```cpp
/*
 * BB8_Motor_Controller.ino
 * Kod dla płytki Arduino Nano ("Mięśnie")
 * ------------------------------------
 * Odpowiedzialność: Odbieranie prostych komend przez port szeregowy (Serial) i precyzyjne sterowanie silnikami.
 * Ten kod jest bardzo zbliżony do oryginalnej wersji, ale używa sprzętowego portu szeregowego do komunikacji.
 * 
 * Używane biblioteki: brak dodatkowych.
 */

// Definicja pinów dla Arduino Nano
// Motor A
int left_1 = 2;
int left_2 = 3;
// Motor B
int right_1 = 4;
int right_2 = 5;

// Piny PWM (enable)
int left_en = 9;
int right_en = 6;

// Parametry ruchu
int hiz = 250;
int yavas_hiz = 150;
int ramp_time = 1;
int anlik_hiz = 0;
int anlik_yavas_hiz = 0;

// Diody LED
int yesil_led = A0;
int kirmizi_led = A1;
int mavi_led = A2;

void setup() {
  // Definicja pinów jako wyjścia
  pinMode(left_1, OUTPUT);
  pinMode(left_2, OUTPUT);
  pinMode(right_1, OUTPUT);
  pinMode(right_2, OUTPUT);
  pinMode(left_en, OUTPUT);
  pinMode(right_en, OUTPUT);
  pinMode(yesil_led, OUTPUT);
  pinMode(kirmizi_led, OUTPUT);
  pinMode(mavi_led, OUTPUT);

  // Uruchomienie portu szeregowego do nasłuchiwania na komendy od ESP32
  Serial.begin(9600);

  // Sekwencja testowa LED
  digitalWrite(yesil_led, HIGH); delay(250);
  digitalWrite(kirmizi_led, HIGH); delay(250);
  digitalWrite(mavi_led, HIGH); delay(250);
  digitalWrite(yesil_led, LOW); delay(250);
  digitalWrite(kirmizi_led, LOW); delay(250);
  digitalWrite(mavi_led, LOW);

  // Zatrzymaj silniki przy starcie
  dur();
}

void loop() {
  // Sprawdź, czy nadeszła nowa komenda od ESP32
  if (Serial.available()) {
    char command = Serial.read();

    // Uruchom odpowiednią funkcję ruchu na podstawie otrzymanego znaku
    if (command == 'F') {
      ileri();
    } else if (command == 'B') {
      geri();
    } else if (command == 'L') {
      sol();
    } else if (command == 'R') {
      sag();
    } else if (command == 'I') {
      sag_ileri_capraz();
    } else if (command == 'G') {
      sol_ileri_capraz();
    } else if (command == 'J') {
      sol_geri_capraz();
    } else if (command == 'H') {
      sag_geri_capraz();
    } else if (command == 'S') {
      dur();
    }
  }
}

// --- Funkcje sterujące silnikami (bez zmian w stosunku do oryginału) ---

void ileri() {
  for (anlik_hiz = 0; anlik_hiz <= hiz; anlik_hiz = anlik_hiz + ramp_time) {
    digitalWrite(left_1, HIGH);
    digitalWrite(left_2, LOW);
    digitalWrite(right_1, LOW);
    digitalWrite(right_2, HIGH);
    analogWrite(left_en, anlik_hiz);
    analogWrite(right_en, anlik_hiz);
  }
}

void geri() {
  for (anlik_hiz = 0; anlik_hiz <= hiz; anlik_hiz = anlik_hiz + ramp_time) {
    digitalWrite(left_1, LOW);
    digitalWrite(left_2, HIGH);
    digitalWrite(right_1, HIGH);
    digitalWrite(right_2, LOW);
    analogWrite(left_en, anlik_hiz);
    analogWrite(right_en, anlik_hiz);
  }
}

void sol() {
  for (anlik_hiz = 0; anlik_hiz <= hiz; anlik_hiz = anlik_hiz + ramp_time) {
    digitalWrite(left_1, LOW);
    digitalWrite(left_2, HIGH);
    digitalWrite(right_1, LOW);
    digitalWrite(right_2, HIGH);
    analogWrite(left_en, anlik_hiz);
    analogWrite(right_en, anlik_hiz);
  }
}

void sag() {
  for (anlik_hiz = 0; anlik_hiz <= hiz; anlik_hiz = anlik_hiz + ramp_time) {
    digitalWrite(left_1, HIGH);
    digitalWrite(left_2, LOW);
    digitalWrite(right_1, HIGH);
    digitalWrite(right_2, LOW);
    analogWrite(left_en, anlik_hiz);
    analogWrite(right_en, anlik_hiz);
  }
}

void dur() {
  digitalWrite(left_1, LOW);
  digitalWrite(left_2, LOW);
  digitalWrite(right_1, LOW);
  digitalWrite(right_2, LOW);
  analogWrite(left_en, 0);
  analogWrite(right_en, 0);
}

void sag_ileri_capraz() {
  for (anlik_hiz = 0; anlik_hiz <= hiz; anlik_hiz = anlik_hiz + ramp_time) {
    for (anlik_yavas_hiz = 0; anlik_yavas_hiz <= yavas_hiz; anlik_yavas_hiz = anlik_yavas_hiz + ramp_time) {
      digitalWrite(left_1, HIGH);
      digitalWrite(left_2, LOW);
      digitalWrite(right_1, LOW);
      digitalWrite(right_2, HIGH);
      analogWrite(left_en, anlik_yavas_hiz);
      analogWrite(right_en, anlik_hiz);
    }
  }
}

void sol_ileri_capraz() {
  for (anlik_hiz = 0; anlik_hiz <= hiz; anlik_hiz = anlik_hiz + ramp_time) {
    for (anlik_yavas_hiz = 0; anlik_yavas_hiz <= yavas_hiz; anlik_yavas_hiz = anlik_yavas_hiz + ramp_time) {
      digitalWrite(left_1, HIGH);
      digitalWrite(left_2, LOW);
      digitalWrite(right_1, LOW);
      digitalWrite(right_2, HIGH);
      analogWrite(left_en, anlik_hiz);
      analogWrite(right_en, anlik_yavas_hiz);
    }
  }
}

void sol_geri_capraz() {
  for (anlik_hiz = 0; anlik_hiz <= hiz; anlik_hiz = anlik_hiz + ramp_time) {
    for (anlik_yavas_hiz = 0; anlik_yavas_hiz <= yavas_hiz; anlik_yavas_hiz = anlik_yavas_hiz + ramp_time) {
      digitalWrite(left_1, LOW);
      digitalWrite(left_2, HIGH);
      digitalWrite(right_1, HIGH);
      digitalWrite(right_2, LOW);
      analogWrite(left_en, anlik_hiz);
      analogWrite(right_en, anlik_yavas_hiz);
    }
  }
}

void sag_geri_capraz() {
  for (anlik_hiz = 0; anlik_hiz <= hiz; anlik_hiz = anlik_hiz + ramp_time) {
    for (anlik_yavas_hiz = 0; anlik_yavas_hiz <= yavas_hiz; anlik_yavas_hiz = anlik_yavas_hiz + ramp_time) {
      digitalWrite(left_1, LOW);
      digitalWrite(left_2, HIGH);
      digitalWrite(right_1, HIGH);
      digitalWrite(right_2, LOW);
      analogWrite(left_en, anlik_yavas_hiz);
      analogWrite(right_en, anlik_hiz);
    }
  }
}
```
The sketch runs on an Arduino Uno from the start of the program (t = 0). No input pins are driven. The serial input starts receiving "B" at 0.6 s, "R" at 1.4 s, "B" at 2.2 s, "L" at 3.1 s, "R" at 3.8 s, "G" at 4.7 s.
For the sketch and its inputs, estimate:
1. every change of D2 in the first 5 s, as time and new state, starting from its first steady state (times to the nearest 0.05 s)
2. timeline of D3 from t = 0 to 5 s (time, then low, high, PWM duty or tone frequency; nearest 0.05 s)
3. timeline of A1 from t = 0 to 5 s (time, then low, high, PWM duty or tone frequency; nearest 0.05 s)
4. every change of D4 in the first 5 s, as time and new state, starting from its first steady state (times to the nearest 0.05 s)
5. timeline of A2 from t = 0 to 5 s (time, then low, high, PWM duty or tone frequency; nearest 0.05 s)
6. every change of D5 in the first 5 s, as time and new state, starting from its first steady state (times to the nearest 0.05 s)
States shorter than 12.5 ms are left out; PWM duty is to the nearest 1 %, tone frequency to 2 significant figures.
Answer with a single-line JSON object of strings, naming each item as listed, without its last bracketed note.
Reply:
{"every change of D2 in the first 5 s, as time and new state, starting from its first steady state": "0 s low; 1.4 s high; 2.2 s low; 3.8 s high", "timeline of D3 from t = 0 to 5 s": "0 s low; 1.25 s high; 1.4 s low; 2.2 s high; 3.8 s low", "timeline of A1 from t = 0 to 5 s": "0 s low; 0.25 s high; 1 s low", "every change of D4 in the first 5 s, as time and new state, starting from its first steady state": "0 s low; 1.25 s high; 3.1 s low; 3.8 s high; 4.7 s low", "timeline of A2 from t = 0 to 5 s": "0 s low; 0.5 s high; 1.25 s low", "every change of D5 in the first 5 s, as time and new state, starting from its first steady state": "0 s low; 3.1 s high; 3.8 s low; 4.7 s high"}
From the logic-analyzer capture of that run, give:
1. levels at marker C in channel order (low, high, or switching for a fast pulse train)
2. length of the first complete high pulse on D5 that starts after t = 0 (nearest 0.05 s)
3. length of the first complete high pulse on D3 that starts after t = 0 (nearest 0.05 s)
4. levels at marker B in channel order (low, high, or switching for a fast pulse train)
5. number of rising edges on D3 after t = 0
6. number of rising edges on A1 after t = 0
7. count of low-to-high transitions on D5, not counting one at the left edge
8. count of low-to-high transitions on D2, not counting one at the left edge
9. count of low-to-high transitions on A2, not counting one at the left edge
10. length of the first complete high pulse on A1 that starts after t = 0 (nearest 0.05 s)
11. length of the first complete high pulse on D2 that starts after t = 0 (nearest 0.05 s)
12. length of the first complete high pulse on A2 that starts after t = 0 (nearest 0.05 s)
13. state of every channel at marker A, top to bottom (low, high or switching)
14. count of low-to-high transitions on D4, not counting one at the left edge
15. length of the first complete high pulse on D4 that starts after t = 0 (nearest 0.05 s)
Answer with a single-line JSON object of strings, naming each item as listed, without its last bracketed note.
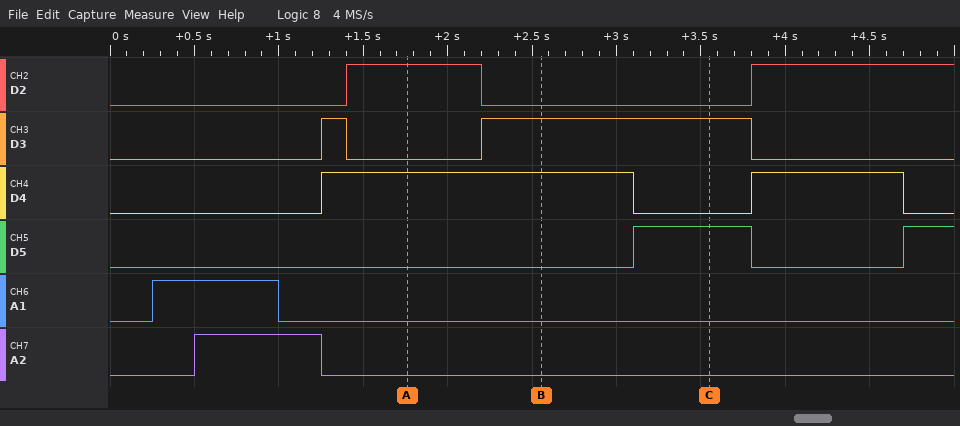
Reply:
{"levels at marker C in channel order": "D2 low, D3 high, D4 low, D5 high, A1 low, A2 low", "length of the first complete high pulse on D5 that starts after t = 0": "0.70 s", "length of the first complete high pulse on D3 that starts after t = 0": "0.15 s", "levels at marker B in channel order": "D2 low, D3 high, D4 high, D5 low, A1 low, A2 low", "number of rising edges on D3 after t = 0": "2", "number of rising edges on A1 after t = 0": "1", "count of low-to-high transitions on D5, not counting one at the left edge": "2", "count of low-to-high transitions on D2, not counting one at the left edge": "2", "count of low-to-high transitions on A2, not counting one at the left edge": "1", "length of the first complete high pulse on A1 that starts after t = 0": "0.75 s", "length of the first complete high pulse on D2 that starts after t = 0": "0.80 s", "length of the first complete high pulse on A2 that starts after t = 0": "0.75 s", "state of every channel at marker A, top to bottom": "D2 high, D3 low, D4 high, D5 low, A1 low, A2 low", "count of low-to-high transitions on D4, not counting one at the left edge": "2", "length of the first complete high pulse on D4 that starts after t = 0": "1.85 s"}
